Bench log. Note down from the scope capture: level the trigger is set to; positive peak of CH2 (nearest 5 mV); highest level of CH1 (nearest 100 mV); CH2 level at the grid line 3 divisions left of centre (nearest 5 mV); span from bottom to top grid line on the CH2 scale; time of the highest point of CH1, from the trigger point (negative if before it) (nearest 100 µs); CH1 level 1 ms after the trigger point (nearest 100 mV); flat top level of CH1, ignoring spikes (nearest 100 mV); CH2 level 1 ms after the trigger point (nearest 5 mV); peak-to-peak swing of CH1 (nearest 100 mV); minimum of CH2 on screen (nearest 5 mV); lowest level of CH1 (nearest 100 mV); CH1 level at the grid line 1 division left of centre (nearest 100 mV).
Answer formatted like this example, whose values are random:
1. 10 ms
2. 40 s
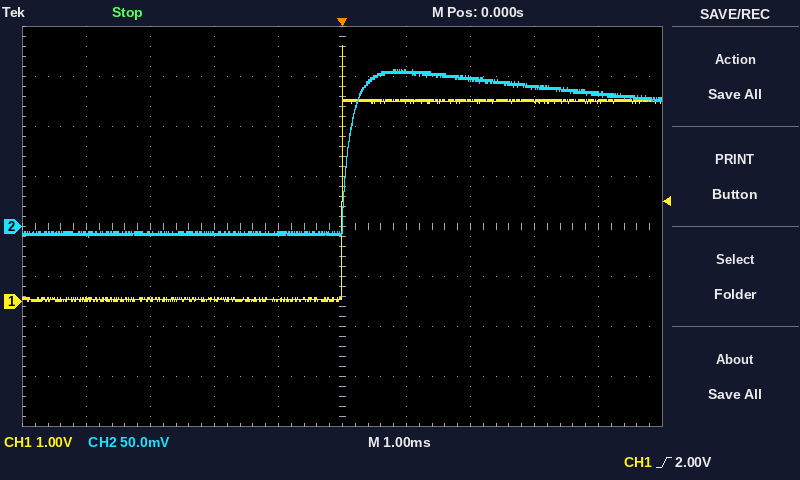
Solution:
1. 2.00 V
2. 155 mV
3. 5.1 V
4. -5 mV
5. 400 mV
6. 0.0 ms
7. 4.0 V
8. 4.0 V
9. 155 mV
10. 5.1 V
11. -10 mV
12. 0.0 V
13. 0.0 V
